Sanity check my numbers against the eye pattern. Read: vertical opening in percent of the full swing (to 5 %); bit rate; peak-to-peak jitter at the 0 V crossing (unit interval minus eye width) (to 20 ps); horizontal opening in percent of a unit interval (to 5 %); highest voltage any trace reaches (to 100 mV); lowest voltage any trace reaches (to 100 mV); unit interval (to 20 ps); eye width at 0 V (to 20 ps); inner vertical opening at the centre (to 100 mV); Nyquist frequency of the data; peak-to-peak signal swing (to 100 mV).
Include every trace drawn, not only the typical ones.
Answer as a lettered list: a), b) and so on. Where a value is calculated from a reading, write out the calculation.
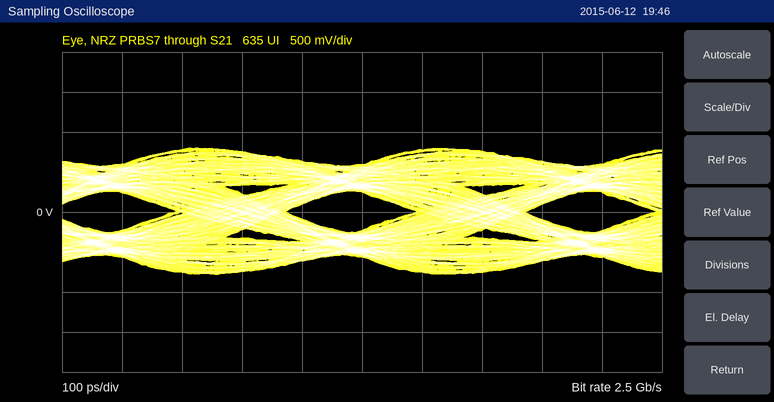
a) 500 mV / 1.6 V ≈ 31.2 %, so 30 % to the nearest 5 %
b) 2.5 Gb/s
c) 180 ps
d) 220 ps / 400 ps ≈ 55 %
e) 800 mV
f) -800 mV
g) 400 ps
h) 220 ps
i) 500 mV
j) 1.25 GHz
k) 1.6 V
